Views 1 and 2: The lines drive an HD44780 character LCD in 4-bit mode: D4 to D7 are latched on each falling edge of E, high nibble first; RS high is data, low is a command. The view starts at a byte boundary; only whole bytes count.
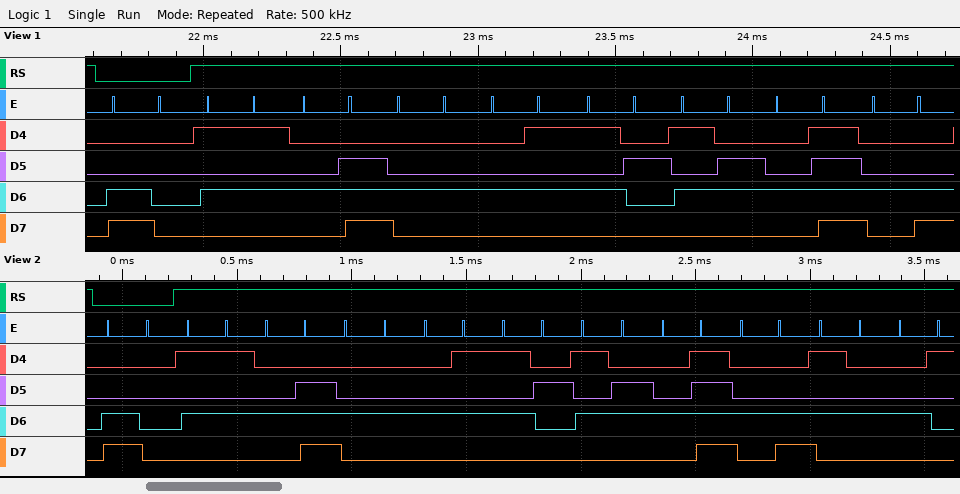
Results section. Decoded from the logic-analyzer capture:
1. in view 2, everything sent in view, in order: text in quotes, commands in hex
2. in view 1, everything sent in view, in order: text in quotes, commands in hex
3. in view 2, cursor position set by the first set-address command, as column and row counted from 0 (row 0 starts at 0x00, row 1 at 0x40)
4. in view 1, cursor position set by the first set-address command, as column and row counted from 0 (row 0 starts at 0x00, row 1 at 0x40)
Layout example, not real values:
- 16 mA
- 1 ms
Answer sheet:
- 0xC0 "UNDERVOLTA"
- 0xC0 "UNDERVOL"
- column 0, row 1
- column 0, row 1
